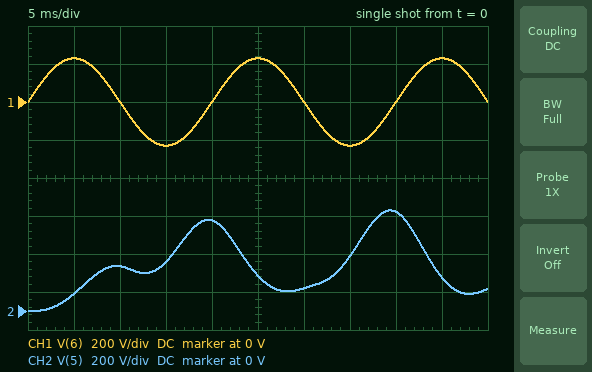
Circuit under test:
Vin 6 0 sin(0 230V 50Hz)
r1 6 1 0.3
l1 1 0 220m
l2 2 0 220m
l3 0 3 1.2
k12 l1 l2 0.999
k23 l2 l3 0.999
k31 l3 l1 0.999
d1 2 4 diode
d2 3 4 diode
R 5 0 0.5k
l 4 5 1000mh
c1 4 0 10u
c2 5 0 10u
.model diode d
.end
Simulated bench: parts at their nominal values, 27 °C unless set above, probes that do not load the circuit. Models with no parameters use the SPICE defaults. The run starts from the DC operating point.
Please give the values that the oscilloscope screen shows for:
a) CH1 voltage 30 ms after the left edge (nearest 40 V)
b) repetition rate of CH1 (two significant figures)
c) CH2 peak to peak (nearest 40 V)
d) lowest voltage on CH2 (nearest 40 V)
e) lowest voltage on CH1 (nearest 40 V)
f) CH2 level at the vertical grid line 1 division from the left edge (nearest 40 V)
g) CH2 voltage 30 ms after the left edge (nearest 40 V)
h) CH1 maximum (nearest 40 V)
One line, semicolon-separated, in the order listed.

0 V; 50 Hz; 520 V; 0 V; -240 V; 80 V; 120 V; 240 V
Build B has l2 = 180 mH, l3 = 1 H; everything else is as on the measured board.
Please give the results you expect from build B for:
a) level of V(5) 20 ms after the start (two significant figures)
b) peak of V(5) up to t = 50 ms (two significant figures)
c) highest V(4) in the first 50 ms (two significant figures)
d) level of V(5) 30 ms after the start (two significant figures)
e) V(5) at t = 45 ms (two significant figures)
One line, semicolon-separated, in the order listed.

440 V; 480 V; 500 V; 110 V; 160 V
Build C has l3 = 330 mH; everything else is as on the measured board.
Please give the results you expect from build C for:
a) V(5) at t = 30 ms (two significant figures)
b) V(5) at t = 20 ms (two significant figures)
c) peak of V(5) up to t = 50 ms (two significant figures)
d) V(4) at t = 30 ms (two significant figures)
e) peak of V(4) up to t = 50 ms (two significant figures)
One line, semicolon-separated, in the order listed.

170 V; 210 V; 240 V; 70 V; 280 V
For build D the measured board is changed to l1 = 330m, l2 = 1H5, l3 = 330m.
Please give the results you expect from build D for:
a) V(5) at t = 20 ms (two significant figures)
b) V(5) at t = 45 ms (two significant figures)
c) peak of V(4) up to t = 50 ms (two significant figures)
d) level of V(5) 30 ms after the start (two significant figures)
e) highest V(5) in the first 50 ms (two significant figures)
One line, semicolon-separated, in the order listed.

120 V; 270 V; 500 V; 470 V; 510 V
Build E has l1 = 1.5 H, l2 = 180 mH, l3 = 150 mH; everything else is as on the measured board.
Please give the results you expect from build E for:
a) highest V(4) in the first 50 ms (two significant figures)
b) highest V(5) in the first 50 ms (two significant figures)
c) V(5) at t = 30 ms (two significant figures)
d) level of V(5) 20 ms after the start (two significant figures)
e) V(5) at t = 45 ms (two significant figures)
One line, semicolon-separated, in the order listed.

79 V; 82 V; 66 V; 48 V; 44 V
